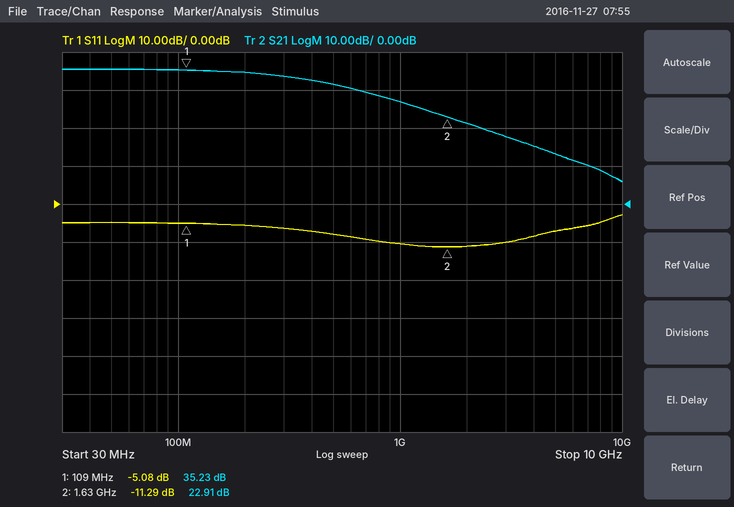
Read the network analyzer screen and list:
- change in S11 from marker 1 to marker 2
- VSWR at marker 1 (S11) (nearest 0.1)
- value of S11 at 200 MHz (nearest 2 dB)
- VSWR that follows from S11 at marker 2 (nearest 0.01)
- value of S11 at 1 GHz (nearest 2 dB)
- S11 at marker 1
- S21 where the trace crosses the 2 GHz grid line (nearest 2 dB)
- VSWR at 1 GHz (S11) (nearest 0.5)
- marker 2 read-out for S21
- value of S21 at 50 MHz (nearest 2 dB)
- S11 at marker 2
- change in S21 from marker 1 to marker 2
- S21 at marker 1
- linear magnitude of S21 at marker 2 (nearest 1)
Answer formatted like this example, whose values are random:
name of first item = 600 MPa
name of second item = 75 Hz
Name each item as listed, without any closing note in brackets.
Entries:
change in S11 from marker 1 to marker 2 = -6.21 dB
VSWR at marker 1 (S11) = 3.5
value of S11 at 200 MHz = -6 dB
VSWR that follows from S11 at marker 2 = 1.75
value of S11 at 1 GHz = -10 dB
S11 at marker 1 = -5.08 dB
S21 where the trace crosses the 2 GHz grid line = 22 dB
VSWR at 1 GHz (S11) = 2.0
marker 2 read-out for S21 = 22.91 dB
value of S21 at 50 MHz = 36 dB
S11 at marker 2 = -11.29 dB
change in S21 from marker 1 to marker 2 = -12.32 dB
S21 at marker 1 = 35.23 dB
linear magnitude of S21 at marker 2 = 14
